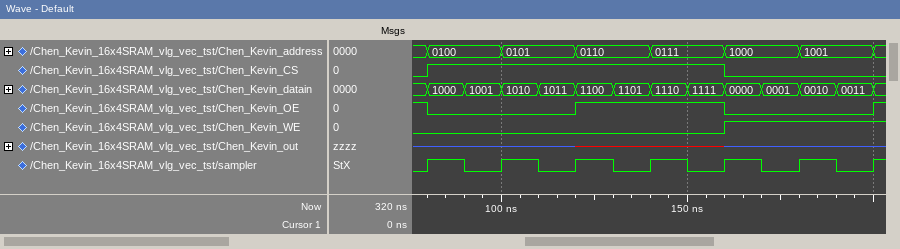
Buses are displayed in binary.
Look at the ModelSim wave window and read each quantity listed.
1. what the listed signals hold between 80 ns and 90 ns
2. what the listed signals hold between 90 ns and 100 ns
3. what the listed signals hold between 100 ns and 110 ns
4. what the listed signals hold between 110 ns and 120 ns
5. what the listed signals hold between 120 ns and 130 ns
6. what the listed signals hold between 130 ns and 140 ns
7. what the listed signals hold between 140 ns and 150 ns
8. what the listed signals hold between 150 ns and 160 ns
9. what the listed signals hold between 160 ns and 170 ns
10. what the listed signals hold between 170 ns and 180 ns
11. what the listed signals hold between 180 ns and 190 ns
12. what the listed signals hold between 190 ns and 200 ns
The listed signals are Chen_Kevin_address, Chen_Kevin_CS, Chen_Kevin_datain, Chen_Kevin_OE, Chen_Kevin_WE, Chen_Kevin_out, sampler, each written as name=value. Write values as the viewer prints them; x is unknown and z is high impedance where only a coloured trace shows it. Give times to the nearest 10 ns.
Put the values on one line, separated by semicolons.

Chen_Kevin_address=0100, Chen_Kevin_CS=1, Chen_Kevin_datain=1000, Chen_Kevin_OE=0, Chen_Kevin_WE=0, Chen_Kevin_out=z, sampler=1; Chen_Kevin_address=0100, Chen_Kevin_CS=1, Chen_Kevin_datain=1001, Chen_Kevin_OE=0, Chen_Kevin_WE=0, Chen_Kevin_out=z, sampler=0; Chen_Kevin_address=0101, Chen_Kevin_CS=1, Chen_Kevin_datain=1010, Chen_Kevin_OE=0, Chen_Kevin_WE=0, Chen_Kevin_out=z, sampler=1; Chen_Kevin_address=0101, Chen_Kevin_CS=1, Chen_Kevin_datain=1011, Chen_Kevin_OE=0, Chen_Kevin_WE=0, Chen_Kevin_out=z, sampler=0; Chen_Kevin_address=0110, Chen_Kevin_CS=1, Chen_Kevin_datain=1100, Chen_Kevin_OE=1, Chen_Kevin_WE=0, Chen_Kevin_out=x, sampler=1; Chen_Kevin_address=0110, Chen_Kevin_CS=1, Chen_Kevin_datain=1101, Chen_Kevin_OE=1, Chen_Kevin_WE=0, Chen_Kevin_out=x, sampler=0; Chen_Kevin_address=0111, Chen_Kevin_CS=1, Chen_Kevin_datain=1110, Chen_Kevin_OE=1, Chen_Kevin_WE=0, Chen_Kevin_out=x, sampler=1; Chen_Kevin_address=0111, Chen_Kevin_CS=1, Chen_Kevin_datain=1111, Chen_Kevin_OE=1, Chen_Kevin_WE=0, Chen_Kevin_out=x, sampler=0; Chen_Kevin_address=1000, Chen_Kevin_CS=0, Chen_Kevin_datain=0000, Chen_Kevin_OE=0, Chen_Kevin_WE=1, Chen_Kevin_out=z, sampler=1; Chen_Kevin_address=1000, Chen_Kevin_CS=0, Chen_Kevin_datain=0001, Chen_Kevin_OE=0, Chen_Kevin_WE=1, Chen_Kevin_out=z, sampler=0; Chen_Kevin_address=1001, Chen_Kevin_CS=0, Chen_Kevin_datain=0010, Chen_Kevin_OE=0, Chen_Kevin_WE=1, Chen_Kevin_out=z, sampler=1; Chen_Kevin_address=1001, Chen_Kevin_CS=0, Chen_Kevin_datain=0011, Chen_Kevin_OE=0, Chen_Kevin_WE=1, Chen_Kevin_out=z, sampler=0
